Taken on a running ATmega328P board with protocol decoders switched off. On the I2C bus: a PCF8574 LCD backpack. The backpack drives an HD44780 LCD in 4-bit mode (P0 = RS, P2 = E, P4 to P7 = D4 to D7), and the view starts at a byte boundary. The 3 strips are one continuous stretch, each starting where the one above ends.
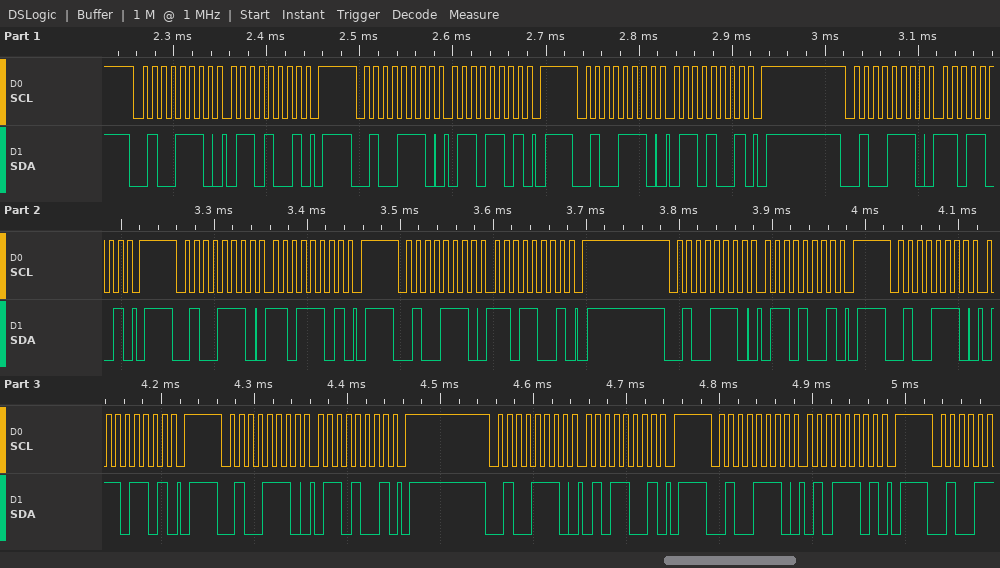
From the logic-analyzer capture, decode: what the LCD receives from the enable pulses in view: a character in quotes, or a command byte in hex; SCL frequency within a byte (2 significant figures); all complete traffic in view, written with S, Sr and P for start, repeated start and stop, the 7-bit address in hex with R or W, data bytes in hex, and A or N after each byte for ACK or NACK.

'm'
100 kHz
S 27W A 69 A P S 27W A 6D A P S 27W A 69 A P S 27W A D9 A P S 27W A DD A P S 27W A D9 A P S 27W A 69 A P S 27W A 6D A P S 27W A 69 A P S 27W A 59 A P S 27W A 5D A P
